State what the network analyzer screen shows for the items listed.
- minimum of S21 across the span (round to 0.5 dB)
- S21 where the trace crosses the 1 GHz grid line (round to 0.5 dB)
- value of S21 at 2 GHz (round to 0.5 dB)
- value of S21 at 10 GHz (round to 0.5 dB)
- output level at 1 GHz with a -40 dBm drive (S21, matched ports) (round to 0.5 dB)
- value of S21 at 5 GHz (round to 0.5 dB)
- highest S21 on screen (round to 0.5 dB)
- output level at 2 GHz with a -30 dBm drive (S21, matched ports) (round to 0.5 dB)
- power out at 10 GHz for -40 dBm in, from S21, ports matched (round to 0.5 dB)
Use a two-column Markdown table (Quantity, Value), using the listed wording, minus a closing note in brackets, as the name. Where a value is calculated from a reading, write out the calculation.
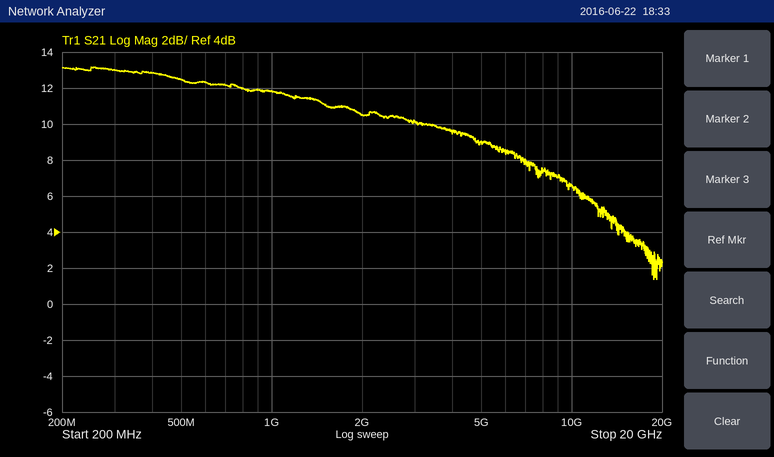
| Quantity | Value |
|---|---|
| minimum of S21 across the span | 1.5 dB |
| S21 where the trace crosses the 1 GHz grid line | 12.0 dB |
| value of S21 at 2 GHz | 10.5 dB |
| value of S21 at 10 GHz | 6.5 dB |
| output level at 1 GHz with a -40 dBm drive (S21, matched ports) | -40 dBm + (12.0 dB) = -28.0 dBm |
| value of S21 at 5 GHz | 9.0 dB |
| highest S21 on screen | 13.0 dB |
| output level at 2 GHz with a -30 dBm drive (S21, matched ports) | -30 dBm + (10.5 dB) = -19.5 dBm |
| power out at 10 GHz for -40 dBm in, from S21, ports matched | -40 dBm + (6.5 dB) = -33.5 dBm |
